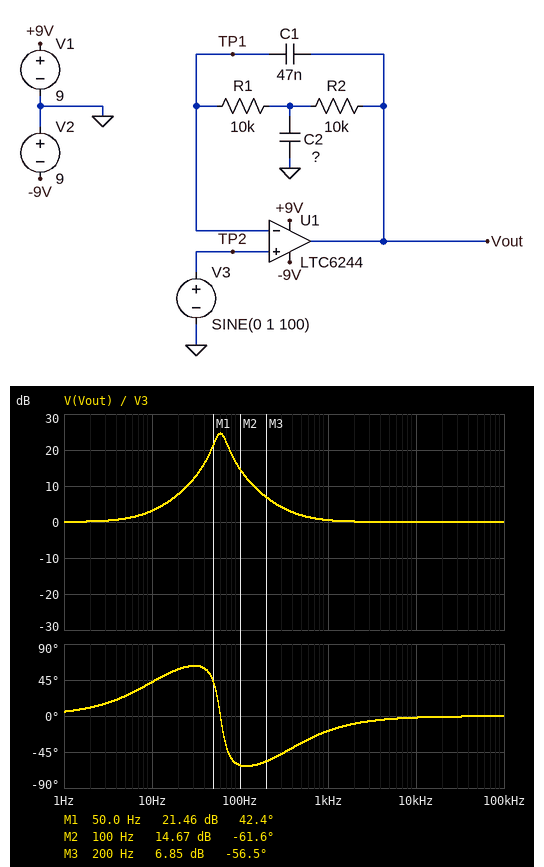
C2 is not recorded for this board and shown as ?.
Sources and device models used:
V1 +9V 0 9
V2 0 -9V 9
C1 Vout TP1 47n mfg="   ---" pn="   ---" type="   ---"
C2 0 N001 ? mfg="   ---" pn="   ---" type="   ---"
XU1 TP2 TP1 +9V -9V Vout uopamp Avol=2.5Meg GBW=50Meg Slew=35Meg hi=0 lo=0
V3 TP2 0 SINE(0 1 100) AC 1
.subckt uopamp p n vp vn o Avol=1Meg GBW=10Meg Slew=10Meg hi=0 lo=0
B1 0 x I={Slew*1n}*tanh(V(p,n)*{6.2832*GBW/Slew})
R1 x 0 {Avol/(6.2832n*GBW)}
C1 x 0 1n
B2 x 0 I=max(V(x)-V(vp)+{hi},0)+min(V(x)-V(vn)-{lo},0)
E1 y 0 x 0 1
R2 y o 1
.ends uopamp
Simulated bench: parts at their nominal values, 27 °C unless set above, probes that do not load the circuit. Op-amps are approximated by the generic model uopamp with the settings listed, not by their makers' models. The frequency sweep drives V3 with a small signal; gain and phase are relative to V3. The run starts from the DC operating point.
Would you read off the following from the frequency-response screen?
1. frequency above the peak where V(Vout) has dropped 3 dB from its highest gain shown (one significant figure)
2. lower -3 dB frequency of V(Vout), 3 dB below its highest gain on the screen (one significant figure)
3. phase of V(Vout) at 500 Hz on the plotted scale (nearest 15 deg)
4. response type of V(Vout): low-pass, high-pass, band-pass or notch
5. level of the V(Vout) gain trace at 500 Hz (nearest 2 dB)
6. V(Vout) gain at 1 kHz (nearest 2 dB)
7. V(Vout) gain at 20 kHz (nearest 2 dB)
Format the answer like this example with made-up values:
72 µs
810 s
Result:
70 Hz
50 Hz
-30 deg
band-pass
2 dB
0 dB
0 dB
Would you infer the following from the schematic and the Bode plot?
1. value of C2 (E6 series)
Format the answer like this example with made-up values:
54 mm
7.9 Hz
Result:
1.5 µF
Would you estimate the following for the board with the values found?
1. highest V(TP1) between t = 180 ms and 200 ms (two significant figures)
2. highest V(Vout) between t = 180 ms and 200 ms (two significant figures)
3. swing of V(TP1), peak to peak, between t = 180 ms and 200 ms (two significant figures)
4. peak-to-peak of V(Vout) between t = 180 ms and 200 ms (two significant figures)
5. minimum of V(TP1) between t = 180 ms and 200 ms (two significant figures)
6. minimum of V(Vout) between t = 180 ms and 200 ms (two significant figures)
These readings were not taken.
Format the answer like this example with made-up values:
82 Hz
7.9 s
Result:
1.0 V
5.4 V
2.0 V
11 V
-1.0 V
-5.4 V
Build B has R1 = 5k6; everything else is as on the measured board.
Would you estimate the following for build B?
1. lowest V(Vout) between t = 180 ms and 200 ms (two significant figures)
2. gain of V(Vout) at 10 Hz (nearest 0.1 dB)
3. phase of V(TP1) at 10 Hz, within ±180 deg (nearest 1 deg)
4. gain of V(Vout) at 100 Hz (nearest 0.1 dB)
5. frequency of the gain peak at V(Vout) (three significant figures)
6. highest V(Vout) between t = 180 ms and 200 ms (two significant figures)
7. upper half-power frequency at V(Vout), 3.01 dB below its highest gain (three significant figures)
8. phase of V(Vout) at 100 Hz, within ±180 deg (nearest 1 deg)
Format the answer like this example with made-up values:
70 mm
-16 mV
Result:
-9.0 V
3.0 dB
0 deg
22.7 dB
80.1 Hz
9.0 V
96.3 Hz
-47 deg
